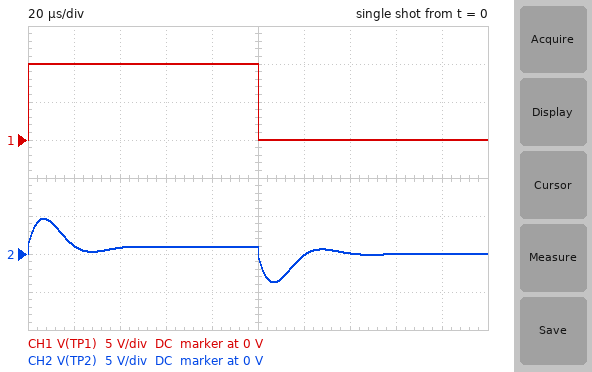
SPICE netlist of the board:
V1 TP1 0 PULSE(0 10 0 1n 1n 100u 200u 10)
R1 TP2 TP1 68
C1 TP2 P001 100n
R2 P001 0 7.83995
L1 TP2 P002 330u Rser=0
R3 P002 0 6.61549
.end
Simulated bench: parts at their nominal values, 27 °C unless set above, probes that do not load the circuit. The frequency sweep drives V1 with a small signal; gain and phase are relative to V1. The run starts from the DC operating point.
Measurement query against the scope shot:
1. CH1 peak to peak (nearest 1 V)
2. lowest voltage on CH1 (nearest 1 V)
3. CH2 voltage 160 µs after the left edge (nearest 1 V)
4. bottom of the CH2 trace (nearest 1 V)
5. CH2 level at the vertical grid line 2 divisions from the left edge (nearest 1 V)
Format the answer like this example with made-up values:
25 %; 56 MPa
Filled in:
10 V; 0 V; 0 V; -4 V; 1 V
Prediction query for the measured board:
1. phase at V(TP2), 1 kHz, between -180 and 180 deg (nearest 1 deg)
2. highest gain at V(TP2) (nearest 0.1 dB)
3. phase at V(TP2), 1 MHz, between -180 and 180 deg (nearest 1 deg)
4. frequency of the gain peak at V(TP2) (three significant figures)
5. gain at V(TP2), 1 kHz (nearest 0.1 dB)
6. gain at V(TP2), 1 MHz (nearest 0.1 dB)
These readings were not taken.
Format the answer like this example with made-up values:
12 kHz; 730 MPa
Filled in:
16 deg; -2.2 dB; -10 deg; 27.5 kHz; -20.6 dB; -19.5 dB
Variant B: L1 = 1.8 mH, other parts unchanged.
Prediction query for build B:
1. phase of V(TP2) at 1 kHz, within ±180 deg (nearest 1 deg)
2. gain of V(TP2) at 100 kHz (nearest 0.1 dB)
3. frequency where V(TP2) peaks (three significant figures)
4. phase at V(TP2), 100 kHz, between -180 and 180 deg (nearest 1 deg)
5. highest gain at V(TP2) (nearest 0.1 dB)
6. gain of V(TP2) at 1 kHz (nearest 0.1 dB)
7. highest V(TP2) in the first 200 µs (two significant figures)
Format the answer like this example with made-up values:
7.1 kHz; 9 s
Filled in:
51 deg; -12.7 dB; 11.8 kHz; -51 deg; -0.5 dB; -15.2 dB; 7.1 V
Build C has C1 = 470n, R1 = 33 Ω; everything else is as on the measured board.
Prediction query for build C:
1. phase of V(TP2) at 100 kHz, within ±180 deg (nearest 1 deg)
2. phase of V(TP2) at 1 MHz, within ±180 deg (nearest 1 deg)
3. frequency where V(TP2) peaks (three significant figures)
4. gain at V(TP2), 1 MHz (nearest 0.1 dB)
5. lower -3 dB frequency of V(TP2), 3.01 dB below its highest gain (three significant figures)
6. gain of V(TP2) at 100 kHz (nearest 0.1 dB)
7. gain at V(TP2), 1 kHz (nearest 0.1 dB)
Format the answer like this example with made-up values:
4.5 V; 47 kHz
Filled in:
-17 deg; -2 deg; 12.7 kHz; -14.3 dB; 7.02 kHz; -13.5 dB; -15.1 dB
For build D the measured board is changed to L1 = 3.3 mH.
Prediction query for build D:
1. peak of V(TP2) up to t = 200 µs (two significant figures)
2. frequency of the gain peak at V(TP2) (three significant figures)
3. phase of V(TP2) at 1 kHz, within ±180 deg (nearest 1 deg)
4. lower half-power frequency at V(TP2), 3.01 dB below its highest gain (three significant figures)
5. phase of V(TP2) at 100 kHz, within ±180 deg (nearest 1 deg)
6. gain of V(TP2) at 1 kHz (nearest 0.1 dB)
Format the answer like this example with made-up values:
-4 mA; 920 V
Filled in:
7.8 V; 8.70 kHz; 56 deg; 3.04 kHz; -52 deg; -10.9 dB
